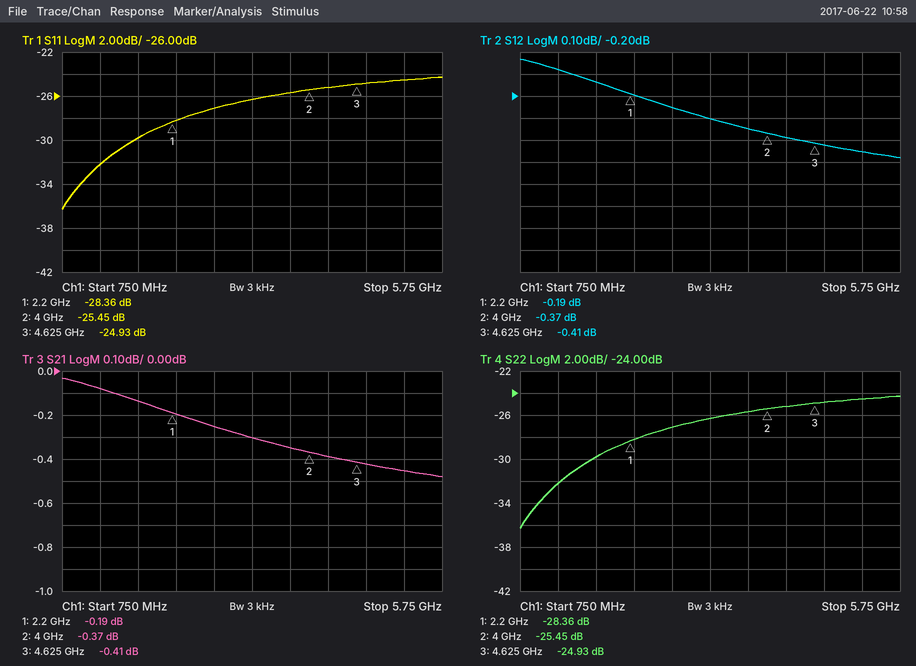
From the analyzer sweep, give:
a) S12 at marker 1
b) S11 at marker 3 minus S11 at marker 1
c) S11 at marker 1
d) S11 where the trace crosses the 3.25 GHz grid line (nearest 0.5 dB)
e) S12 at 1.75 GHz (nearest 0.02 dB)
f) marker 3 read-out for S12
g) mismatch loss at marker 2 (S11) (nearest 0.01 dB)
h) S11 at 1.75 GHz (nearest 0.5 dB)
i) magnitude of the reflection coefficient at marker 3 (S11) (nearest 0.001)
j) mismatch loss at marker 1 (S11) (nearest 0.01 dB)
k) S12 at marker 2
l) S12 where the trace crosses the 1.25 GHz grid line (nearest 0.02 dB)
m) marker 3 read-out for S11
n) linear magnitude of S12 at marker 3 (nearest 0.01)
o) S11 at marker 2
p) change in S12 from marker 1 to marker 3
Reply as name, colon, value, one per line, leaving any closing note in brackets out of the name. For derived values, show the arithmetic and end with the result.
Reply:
S12 at marker 1: -0.19 dB
S11 at marker 3 minus S11 at marker 1: -24.93 − (-28.36) = 3.43 dB
S11 at marker 1: -28.36 dB
S11 where the trace crosses the 3.25 GHz grid line: -26.5 dB
S12 at 1.75 GHz: -0.14 dB
marker 3 read-out for S12: -0.41 dB
mismatch loss at marker 2 (S11): −10 log10(1 − 10^(-25.45/10)) ≈ 0.01 dB
S11 at 1.75 GHz: -30.0 dB
magnitude of the reflection coefficient at marker 3 (S11): 10^(-24.93/20) ≈ 0.057
mismatch loss at marker 1 (S11): −10 log10(1 − 10^(-28.36/10)) ≈ 0.01 dB
S12 at marker 2: -0.37 dB
S12 where the trace crosses the 1.25 GHz grid line: -0.08 dB
marker 3 read-out for S11: -24.93 dB
linear magnitude of S12 at marker 3: 10^(-0.41/20) ≈ 0.95
S11 at marker 2: -25.45 dB
change in S12 from marker 1 to marker 3: -0.41 − (-0.19) = -0.22 dB
